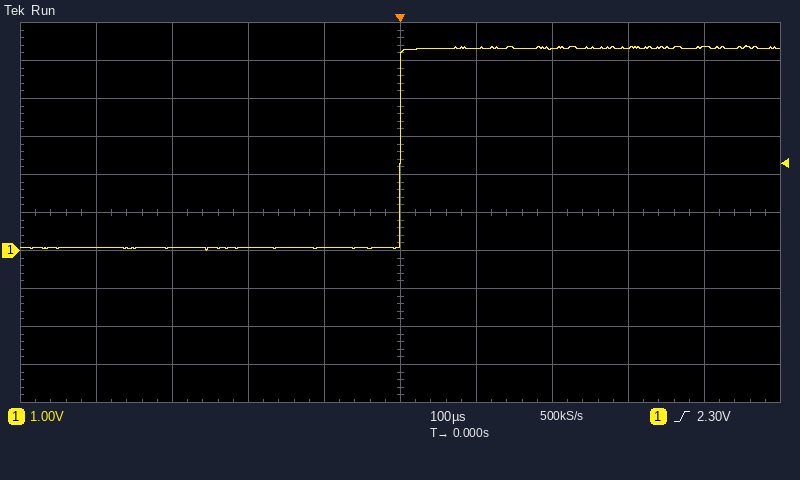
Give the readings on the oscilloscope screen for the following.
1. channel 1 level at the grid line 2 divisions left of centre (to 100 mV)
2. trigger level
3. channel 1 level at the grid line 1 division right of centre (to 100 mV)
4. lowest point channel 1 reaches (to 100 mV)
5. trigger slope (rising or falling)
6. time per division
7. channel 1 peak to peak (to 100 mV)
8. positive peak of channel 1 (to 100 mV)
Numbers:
100 mV
2.30 V
5.3 V
0.0 V
rising
100 µs
5.4 V
5.4 V
